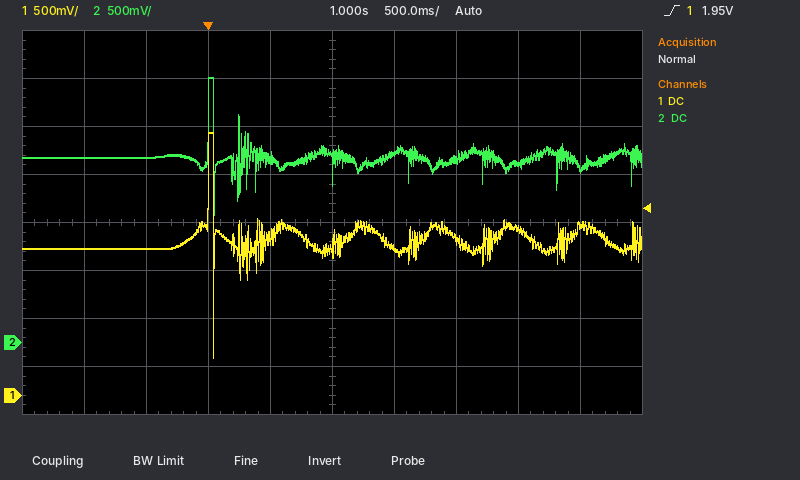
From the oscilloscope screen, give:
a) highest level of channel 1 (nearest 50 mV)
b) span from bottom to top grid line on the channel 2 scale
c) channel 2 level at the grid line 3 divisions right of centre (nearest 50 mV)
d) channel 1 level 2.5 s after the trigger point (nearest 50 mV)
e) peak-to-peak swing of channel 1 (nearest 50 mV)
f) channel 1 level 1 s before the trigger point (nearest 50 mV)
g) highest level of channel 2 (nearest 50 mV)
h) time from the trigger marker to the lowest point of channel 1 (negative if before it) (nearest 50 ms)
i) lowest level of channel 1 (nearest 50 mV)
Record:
2.75 V
4 V
1.85 V
1.75 V
2.35 V
1.55 V
2.75 V
+50 ms
400 mV
